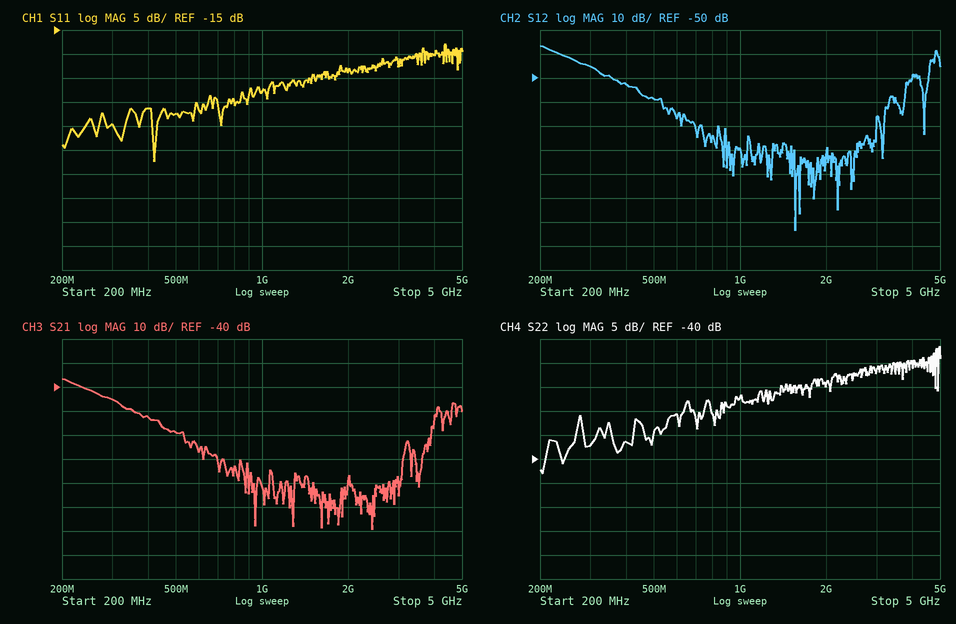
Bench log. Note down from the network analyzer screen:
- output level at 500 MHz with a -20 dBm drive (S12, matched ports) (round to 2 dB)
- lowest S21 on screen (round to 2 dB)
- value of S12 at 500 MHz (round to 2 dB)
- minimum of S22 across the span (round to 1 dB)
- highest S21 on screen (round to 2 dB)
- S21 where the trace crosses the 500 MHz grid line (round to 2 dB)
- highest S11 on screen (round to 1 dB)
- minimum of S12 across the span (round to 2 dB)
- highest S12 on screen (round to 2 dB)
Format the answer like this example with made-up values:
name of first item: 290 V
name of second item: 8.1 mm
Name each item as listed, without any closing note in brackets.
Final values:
output level at 500 MHz with a -20 dBm drive (S12, matched ports): -78 dBm
lowest S21 on screen: -100 dB
value of S12 at 500 MHz: -58 dB
minimum of S22 across the span: -43 dB
highest S21 on screen: -36 dB
S21 where the trace crosses the 500 MHz grid line: -58 dB
highest S11 on screen: -18 dB
minimum of S12 across the span: -114 dB
highest S12 on screen: -36 dB
